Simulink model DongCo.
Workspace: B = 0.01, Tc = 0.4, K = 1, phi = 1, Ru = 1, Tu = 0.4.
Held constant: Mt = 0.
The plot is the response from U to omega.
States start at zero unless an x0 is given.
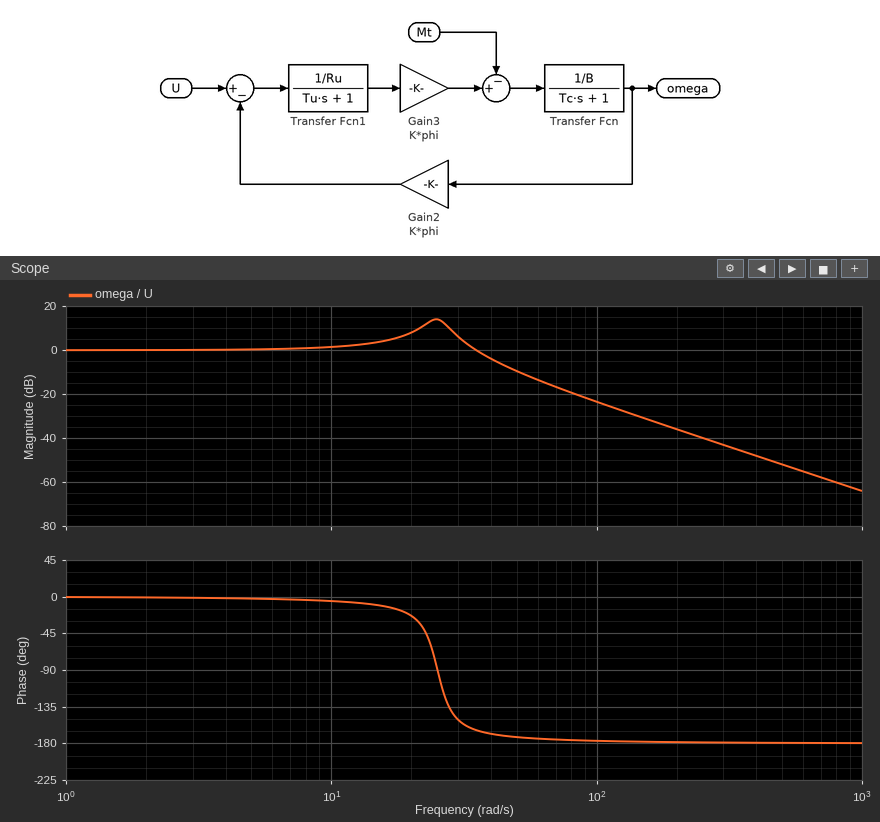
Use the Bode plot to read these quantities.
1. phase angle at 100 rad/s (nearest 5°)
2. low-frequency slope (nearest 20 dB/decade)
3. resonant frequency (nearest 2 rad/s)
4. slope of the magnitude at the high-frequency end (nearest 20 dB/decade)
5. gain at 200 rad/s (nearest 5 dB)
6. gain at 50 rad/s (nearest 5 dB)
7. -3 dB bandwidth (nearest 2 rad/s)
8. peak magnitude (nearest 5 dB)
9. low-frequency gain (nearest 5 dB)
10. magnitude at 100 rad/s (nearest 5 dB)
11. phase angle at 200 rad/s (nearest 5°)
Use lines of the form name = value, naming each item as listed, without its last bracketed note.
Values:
phase angle at 100 rad/s = -175°
low-frequency slope = 0 dB/decade
resonant frequency = 24 rad/s
slope of the magnitude at the high-frequency end = -40 dB/decade
gain at 200 rad/s = -35 dB
gain at 50 rad/s = -10 dB
-3 dB bandwidth = 38 rad/s
peak magnitude = 15 dB
low-frequency gain = 0 dB
magnitude at 100 rad/s = -25 dB
phase angle at 200 rad/s = -180°
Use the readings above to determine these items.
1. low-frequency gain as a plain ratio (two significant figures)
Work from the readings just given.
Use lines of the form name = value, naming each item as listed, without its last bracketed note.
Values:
low-frequency gain as a plain ratio = 1.0
